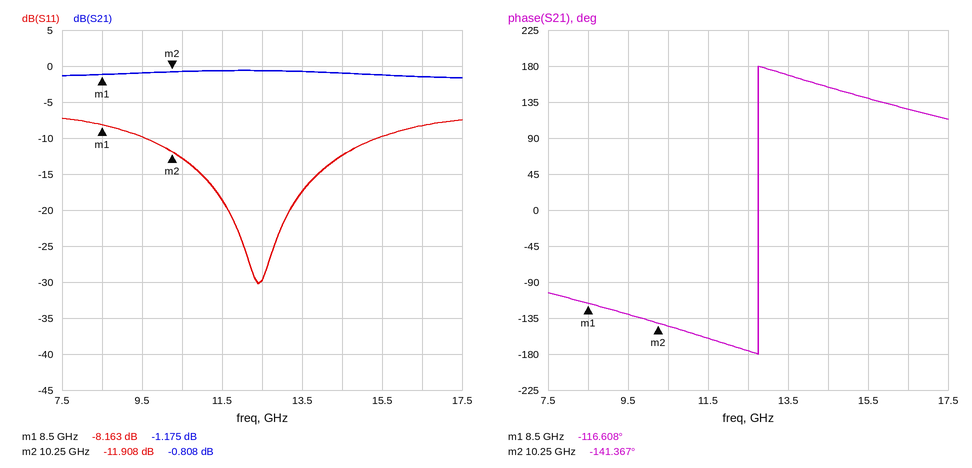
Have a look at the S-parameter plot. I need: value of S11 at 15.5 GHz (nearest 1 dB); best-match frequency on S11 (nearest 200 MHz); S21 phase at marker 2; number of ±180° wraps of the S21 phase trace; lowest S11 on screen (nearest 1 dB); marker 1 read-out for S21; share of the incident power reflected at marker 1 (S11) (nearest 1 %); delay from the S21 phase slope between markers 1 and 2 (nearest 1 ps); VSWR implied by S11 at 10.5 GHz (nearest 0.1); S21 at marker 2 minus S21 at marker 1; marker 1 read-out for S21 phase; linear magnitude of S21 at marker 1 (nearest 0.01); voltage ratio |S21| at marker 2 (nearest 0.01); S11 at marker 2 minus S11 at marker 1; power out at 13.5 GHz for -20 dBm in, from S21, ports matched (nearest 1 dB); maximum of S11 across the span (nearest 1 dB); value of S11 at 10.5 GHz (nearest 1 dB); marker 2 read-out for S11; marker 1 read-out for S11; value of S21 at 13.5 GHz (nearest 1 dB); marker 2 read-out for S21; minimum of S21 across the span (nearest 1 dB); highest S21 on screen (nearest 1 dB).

-10 dB
12.4 GHz
-141.367°
1
-30 dB
-1.175 dB
15 %
39 ps
1.6
0.367 dB
-116.608°
0.87
0.91
-3.745 dB
-21 dBm
-7 dB
-13 dB
-11.908 dB
-8.163 dB
-1 dB
-0.808 dB
-2 dB
-1 dB
